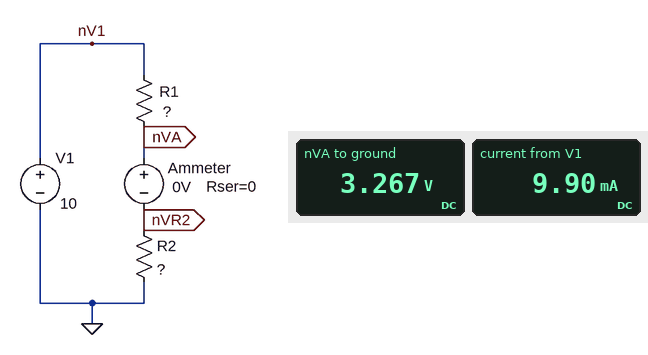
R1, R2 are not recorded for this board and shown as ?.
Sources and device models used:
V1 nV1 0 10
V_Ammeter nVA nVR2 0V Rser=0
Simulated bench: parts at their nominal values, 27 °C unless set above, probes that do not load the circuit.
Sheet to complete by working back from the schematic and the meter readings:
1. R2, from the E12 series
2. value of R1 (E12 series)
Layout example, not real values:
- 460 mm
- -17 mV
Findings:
- 330 Ω
- 680 Ω
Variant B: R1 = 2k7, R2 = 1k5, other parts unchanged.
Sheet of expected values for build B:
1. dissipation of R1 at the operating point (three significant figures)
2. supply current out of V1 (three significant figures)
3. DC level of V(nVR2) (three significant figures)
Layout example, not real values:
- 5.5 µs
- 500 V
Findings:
- 15.3 mW
- 2.38 mA
- 3.57 V
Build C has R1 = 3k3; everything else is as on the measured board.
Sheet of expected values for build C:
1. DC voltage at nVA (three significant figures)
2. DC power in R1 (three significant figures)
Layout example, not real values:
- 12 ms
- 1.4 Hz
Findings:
- 909 mV
- 25.0 mW
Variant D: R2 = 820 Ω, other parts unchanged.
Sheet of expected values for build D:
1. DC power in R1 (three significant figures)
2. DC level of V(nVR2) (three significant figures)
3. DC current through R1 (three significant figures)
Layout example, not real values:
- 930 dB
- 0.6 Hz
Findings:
- 30.2 mW
- 5.47 V
- 6.67 mA
